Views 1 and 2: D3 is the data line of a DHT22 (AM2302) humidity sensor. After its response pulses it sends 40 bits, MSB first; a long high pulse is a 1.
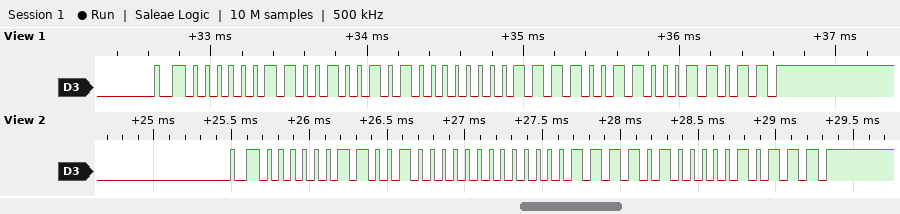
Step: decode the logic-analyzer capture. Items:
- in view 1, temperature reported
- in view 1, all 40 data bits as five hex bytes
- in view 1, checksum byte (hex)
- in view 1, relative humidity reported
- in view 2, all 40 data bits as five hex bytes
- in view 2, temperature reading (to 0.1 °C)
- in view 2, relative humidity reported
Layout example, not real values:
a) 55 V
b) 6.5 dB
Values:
a) 24.3 °C
b) 03 25 00 F3 1B
c) 0x1B
d) 80.5 %
e) 03 20 00 F4 17
f) 24.4 °C
g) 80.0 %
